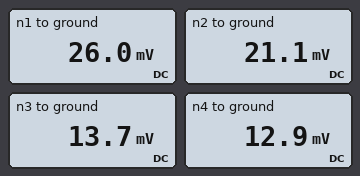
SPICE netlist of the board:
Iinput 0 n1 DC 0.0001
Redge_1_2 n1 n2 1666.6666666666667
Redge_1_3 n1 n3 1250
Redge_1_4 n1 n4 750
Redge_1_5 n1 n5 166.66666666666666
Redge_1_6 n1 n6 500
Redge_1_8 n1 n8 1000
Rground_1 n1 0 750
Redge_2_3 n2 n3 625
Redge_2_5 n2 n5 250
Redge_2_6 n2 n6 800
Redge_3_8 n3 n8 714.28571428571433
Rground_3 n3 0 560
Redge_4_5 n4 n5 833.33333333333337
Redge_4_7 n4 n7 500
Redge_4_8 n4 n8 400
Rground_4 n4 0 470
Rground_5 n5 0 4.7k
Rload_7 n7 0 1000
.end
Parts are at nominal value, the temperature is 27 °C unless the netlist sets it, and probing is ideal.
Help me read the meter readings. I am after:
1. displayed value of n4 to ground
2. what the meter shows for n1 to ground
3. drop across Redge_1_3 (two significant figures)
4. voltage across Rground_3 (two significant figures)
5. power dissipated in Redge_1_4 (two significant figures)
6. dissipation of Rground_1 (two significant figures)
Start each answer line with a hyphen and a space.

- 12.9 mV
- 26.0 mV
- 12 mV
- 14 mV
- 230 nW
- 900 nW
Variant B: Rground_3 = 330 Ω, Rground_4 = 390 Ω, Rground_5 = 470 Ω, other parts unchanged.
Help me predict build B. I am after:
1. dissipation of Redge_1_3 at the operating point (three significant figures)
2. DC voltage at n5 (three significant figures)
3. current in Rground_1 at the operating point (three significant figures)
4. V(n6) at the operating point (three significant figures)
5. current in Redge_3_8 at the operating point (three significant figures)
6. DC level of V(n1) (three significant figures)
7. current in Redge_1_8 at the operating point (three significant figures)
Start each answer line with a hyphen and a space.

- 106 nW
- 13.0 mV
- 25.0 µA
- 16.4 mV
- 3.78 µA
- 18.7 mV
- 8.81 µA
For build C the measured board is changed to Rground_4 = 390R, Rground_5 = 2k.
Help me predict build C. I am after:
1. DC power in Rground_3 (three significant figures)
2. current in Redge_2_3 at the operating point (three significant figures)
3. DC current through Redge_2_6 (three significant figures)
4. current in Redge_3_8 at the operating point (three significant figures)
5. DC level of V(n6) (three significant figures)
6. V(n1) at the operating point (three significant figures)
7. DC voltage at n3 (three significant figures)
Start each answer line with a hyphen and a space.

- 276 nW
- 10.6 µA
- 3.85 µA
- 2.33 µA
- 22.1 mV
- 24.1 mV
- 12.4 mV
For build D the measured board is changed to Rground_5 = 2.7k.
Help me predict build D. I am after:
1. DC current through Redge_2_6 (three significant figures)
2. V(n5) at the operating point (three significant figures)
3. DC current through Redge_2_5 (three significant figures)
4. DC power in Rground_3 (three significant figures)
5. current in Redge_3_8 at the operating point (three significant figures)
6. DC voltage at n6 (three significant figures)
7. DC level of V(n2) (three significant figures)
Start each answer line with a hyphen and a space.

- 3.81 µA
- 21.4 mV
- 4.44 µA
- 313 nW
- 2.85 µA
- 23.3 mV
- 20.3 mV
